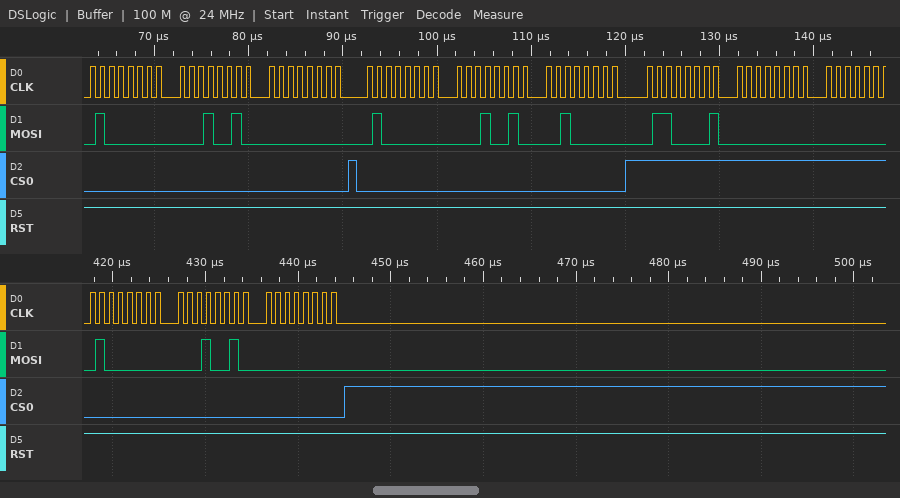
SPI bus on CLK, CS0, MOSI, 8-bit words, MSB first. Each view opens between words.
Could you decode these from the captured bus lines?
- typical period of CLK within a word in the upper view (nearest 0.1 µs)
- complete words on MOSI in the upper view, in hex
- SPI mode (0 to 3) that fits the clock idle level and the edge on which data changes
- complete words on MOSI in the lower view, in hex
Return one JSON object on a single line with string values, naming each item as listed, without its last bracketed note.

{"typical period of CLK within a word in the upper view": "1 µs", "complete words on MOSI in the upper view, in hex": "40, 12, 00, 40, 12, 20, 61, 00", "SPI mode (0 to 3) that fits the clock idle level and the edge on which data changes": "0", "complete words on MOSI in the lower view, in hex": "40, 12, 00"}
